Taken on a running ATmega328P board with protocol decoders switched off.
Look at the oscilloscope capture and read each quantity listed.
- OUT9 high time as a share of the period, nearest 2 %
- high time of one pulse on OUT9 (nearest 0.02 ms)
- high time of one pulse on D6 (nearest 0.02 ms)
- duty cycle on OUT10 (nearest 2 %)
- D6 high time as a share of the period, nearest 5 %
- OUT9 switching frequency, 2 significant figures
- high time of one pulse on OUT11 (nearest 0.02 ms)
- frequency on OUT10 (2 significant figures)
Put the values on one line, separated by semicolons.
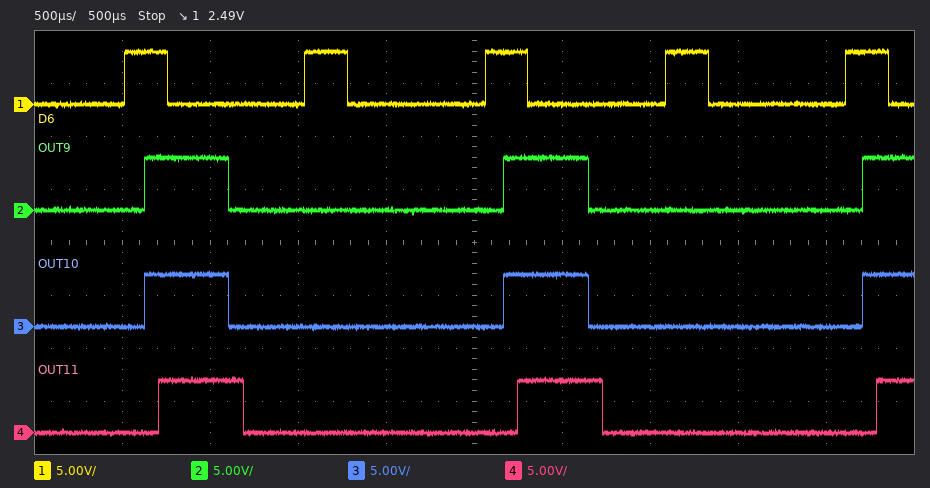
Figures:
24 %; 0.48 ms; 0.24 ms; 24 %; 25 %; 490 Hz; 0.48 ms; 490 Hz
